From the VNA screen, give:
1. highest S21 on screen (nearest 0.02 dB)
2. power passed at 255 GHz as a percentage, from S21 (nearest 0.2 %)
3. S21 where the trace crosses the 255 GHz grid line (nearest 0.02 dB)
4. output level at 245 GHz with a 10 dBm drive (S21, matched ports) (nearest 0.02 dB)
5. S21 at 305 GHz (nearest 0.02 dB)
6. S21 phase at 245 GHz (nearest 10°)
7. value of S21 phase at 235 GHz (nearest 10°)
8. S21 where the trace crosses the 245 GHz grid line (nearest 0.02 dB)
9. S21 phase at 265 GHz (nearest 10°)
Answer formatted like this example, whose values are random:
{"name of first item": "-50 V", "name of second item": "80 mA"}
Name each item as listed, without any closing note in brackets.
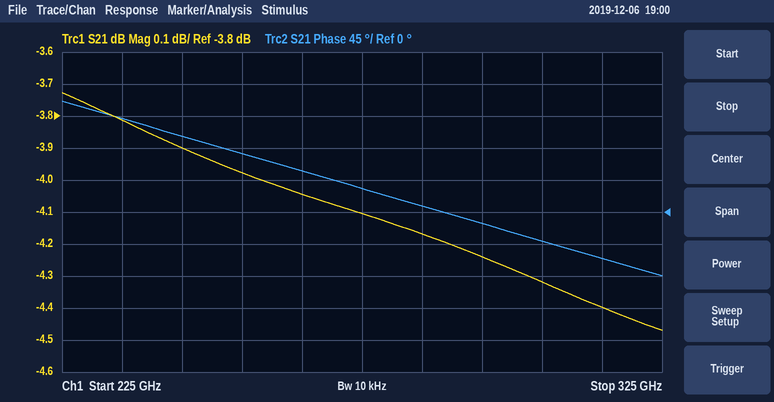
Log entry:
{"highest S21 on screen": "-3.72 dB", "power passed at 255 GHz as a percentage, from S21": "40.0 %", "S21 where the trace crosses the 255 GHz grid line": "-3.98 dB", "output level at 245 GHz with a 10 dBm drive (S21, matched ports)": "6.10 dBm", "S21 at 305 GHz": "-4.32 dB", "S21 phase at 245 GHz": "110°", "value of S21 phase at 235 GHz": "130°", "S21 where the trace crosses the 245 GHz grid line": "-3.90 dB", "S21 phase at 265 GHz": "60°"}
